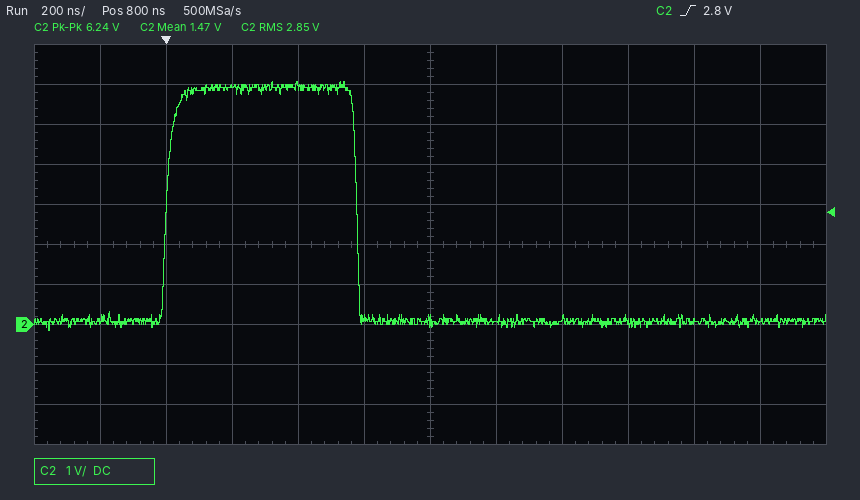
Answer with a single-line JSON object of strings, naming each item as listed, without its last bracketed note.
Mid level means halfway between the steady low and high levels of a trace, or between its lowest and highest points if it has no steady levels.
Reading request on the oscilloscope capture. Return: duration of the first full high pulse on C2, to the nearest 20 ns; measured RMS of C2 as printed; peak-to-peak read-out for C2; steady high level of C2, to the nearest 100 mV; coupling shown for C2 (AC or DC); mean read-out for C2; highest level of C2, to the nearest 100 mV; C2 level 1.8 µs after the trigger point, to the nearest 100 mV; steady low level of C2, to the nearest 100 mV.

{"duration of the first full high pulse on C2, to the nearest 20 ns": "580 ns", "measured RMS of C2 as printed": "2.85 V", "peak-to-peak read-out for C2": "6.24 V", "steady high level of C2, to the nearest 100 mV": "5.9 V", "coupling shown for C2": "DC", "mean read-out for C2": "1.47 V", "highest level of C2, to the nearest 100 mV": "6.1 V", "C2 level 1.8 µs after the trigger point, to the nearest 100 mV": "100 mV", "steady low level of C2, to the nearest 100 mV": "100 mV"}
